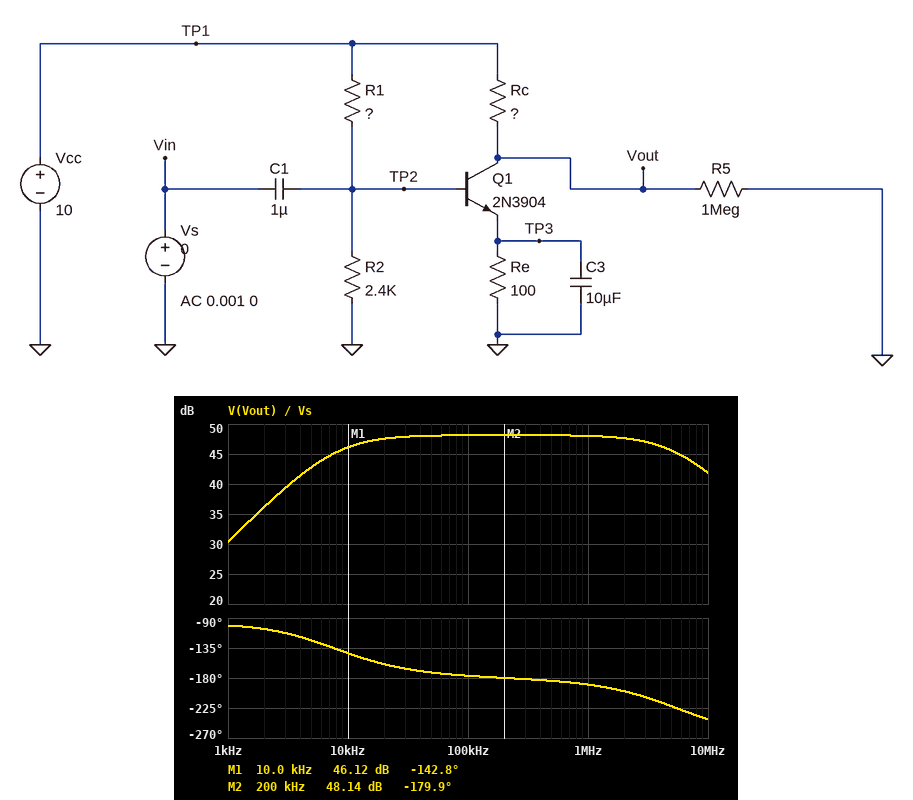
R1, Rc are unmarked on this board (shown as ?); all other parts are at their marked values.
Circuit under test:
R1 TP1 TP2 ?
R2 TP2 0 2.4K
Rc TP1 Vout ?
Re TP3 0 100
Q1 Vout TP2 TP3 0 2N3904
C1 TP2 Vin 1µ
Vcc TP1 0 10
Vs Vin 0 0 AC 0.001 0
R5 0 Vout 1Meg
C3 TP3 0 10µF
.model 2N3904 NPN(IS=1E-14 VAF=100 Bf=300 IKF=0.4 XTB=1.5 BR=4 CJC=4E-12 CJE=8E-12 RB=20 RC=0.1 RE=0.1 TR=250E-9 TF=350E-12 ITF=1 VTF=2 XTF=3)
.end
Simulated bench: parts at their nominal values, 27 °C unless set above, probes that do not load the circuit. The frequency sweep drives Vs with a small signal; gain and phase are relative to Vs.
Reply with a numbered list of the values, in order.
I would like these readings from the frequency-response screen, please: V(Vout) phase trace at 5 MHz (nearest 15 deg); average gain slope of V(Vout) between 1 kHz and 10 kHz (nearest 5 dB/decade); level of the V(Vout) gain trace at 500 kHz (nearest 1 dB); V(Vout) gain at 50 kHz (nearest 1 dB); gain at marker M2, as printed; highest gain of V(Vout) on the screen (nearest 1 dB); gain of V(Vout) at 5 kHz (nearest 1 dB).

1. -225 deg
2. 15 dB/decade
3. 48 dB
4. 48 dB
5. 48.14 dB
6. 48 dB
7. 43 dB
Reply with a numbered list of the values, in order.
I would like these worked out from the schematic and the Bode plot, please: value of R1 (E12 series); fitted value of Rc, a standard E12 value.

1. 8.2 kΩ
2. 560 Ω
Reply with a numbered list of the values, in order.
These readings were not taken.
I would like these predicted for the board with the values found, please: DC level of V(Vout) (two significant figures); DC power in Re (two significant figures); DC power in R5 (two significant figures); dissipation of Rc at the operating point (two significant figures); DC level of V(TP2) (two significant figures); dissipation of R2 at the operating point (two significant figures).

1. 1.9 V
2. 21 mW
3. 3.8 µW
4. 120 mW
5. 2.2 V
6. 2.0 mW
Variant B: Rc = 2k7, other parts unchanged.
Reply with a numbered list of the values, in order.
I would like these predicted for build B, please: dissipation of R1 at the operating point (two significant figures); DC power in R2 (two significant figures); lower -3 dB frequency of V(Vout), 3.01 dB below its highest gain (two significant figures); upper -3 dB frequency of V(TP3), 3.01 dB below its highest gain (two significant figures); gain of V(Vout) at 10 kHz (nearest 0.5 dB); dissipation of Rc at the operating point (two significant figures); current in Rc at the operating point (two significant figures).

1. 9.6 mW
2. 530 µW
3. 4.3 kHz
4. 4.8 kHz
5. -5.5 dB
6. 34 mW
7. 3.5 mA
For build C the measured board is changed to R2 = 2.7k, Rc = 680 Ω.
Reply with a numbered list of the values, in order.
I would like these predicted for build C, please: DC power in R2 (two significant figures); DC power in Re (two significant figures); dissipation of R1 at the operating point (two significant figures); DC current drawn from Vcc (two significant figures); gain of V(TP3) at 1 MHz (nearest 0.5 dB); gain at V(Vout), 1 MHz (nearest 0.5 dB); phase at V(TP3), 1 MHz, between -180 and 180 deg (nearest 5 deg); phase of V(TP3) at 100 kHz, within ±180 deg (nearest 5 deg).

1. 1.5 mW
2. 17 mW
3. 7.8 mW
4. 14 mA
5. -63.0 dB
6. -0.5 dB
7. -90 deg
8. -85 deg
